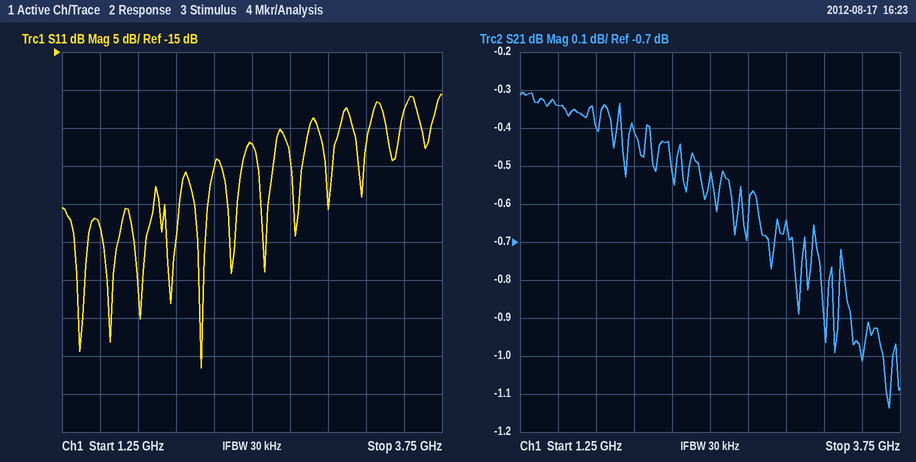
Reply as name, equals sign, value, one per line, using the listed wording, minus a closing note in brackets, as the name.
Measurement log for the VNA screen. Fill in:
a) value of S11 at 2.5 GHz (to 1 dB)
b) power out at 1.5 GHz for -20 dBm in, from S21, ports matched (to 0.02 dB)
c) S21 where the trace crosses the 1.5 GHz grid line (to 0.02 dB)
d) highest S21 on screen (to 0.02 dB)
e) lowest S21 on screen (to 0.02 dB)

value of S11 at 2.5 GHz = -27 dB
power out at 1.5 GHz for -20 dBm in, from S21, ports matched = -20.34 dBm
S21 where the trace crosses the 1.5 GHz grid line = -0.34 dB
highest S21 on screen = -0.30 dB
lowest S21 on screen = -1.14 dB
